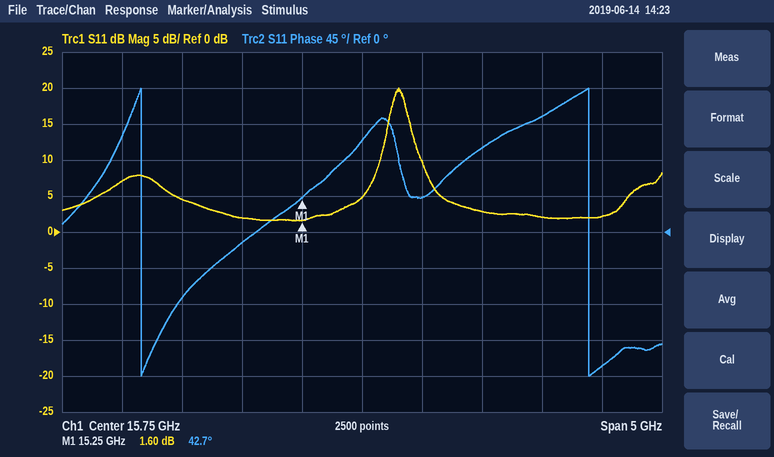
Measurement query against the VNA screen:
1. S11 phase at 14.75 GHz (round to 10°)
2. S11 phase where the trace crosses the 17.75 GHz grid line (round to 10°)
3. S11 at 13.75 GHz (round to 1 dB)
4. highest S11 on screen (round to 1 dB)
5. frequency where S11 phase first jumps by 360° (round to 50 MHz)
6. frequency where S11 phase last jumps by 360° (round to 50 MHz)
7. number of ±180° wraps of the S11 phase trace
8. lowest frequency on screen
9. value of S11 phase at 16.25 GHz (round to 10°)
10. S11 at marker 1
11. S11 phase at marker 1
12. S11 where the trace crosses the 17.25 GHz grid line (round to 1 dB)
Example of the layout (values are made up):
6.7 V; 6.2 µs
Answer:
-10°; -170°; 7 dB; 20 dB; 13.90 GHz; 17.65 GHz; 2; 13.25 GHz; 40°; 1.60 dB; 42.7°; 2 dB
